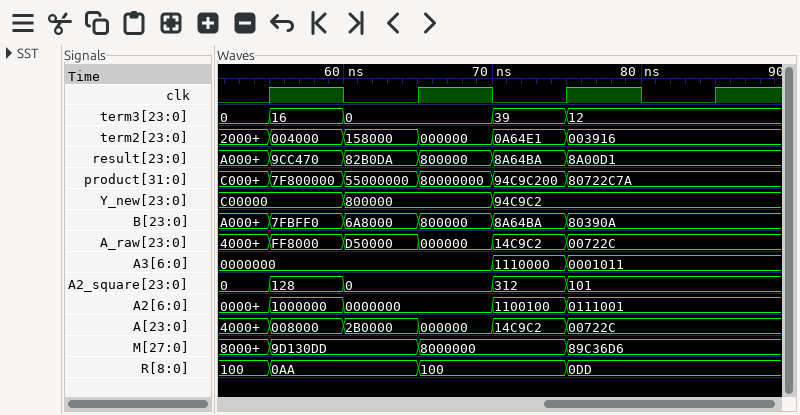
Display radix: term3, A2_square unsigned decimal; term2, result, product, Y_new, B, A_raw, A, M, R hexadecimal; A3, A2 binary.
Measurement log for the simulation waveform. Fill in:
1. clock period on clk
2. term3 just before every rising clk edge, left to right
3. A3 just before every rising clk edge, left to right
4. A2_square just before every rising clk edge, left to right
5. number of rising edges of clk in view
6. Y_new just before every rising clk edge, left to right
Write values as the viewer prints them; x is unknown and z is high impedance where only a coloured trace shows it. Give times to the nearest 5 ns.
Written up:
10 ns
0, 0, 39, 12
0000000, 0000000, 1110000, 0001011
0, 0, 312, 101
4
C00000, 800000, 94C9C2, 94C9C2
